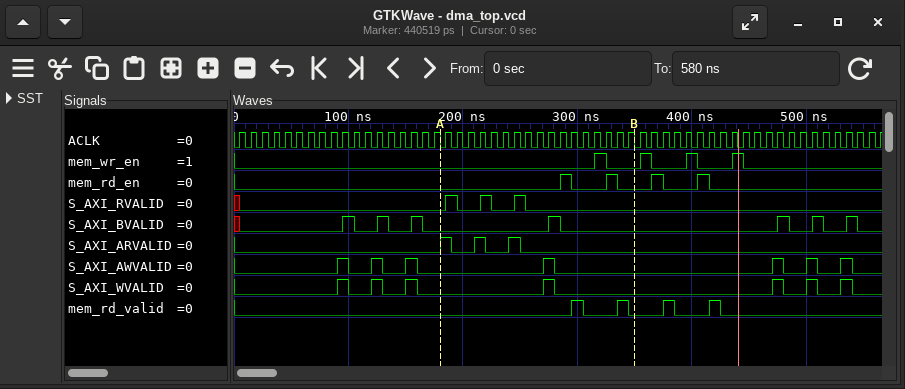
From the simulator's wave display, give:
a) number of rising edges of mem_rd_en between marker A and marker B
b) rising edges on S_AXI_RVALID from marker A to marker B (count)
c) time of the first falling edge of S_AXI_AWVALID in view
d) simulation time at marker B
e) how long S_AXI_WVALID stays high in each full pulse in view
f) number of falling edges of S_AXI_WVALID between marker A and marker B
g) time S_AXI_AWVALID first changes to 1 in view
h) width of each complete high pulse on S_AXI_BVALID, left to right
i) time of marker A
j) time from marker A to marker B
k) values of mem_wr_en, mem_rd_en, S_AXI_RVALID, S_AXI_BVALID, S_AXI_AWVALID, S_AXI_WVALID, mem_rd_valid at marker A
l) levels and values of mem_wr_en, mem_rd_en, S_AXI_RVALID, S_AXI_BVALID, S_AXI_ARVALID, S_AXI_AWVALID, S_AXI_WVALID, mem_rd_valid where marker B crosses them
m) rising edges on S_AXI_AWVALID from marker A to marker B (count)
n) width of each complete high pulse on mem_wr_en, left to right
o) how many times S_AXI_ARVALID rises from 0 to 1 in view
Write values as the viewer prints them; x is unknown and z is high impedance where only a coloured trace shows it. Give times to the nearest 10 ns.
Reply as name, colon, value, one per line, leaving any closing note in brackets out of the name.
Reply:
number of rising edges of mem_rd_en between marker A and marker B: 2
rising edges on S_AXI_RVALID from marker A to marker B: 3
time of the first falling edge of S_AXI_AWVALID in view: 100 ns
simulation time at marker B: 350 ns
how long S_AXI_WVALID stays high in each full pulse in view: 10 ns, 10 ns, 10 ns, 10 ns, 10 ns, 10 ns, 10 ns
number of falling edges of S_AXI_WVALID between marker A and marker B: 1
time S_AXI_AWVALID first changes to 1 in view: 90 ns
width of each complete high pulse on S_AXI_BVALID, left to right: 10 ns, 10 ns, 10 ns, 10 ns, 10 ns, 10 ns, 10 ns
time of marker A: 180 ns
time from marker A to marker B: 170 ns
values of mem_wr_en, mem_rd_en, S_AXI_RVALID, S_AXI_BVALID, S_AXI_AWVALID, S_AXI_WVALID, mem_rd_valid at marker A: mem_wr_en=0, mem_rd_en=0, S_AXI_RVALID=0, S_AXI_BVALID=0, S_AXI_AWVALID=0, S_AXI_WVALID=0, mem_rd_valid=0
levels and values of mem_wr_en, mem_rd_en, S_AXI_RVALID, S_AXI_BVALID, S_AXI_ARVALID, S_AXI_AWVALID, S_AXI_WVALID, mem_rd_valid where marker B crosses them: mem_wr_en=0, mem_rd_en=0, S_AXI_RVALID=0, S_AXI_BVALID=0, S_AXI_ARVALID=0, S_AXI_AWVALID=0, S_AXI_WVALID=0, mem_rd_valid=0
rising edges on S_AXI_AWVALID from marker A to marker B: 1
width of each complete high pulse on mem_wr_en, left to right: 10 ns, 10 ns, 10 ns, 10 ns
how many times S_AXI_ARVALID rises from 0 to 1 in view: 3
